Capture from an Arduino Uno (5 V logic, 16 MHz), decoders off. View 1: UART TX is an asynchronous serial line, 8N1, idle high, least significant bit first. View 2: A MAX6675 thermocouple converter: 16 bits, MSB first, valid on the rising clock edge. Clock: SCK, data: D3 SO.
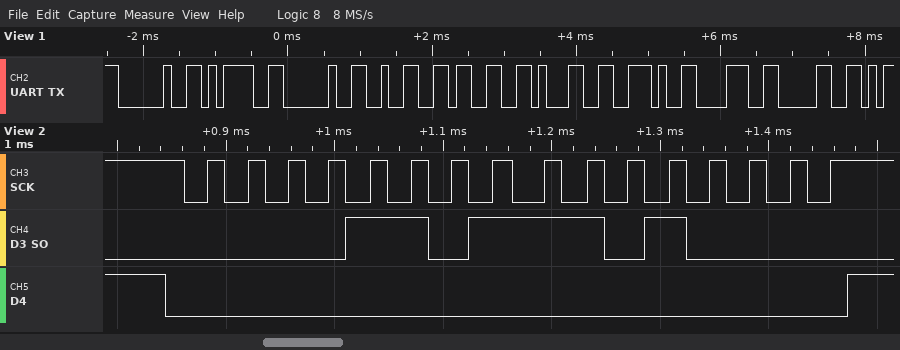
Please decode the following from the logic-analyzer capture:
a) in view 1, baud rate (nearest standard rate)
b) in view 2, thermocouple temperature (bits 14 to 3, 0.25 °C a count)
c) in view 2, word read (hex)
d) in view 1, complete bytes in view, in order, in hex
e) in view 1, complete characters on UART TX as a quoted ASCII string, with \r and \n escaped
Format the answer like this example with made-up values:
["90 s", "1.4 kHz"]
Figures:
["9600 baud", "110.50 °C", "0x0DD0", "20 3D 20 32 33 31 2E 38 30", "\" = 231.80\""]
